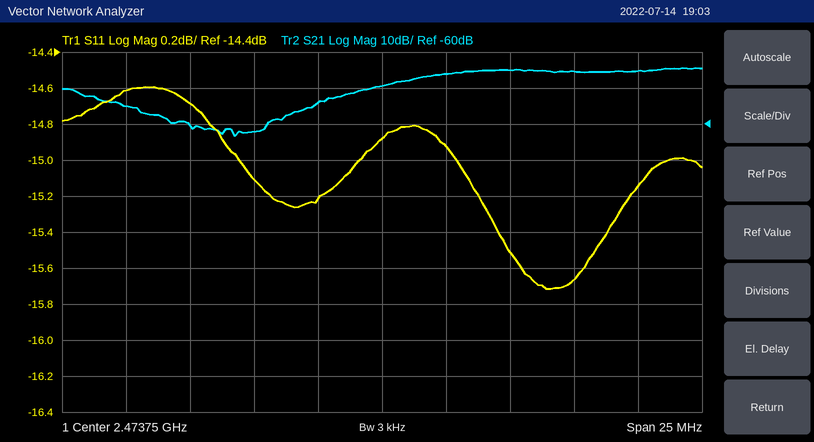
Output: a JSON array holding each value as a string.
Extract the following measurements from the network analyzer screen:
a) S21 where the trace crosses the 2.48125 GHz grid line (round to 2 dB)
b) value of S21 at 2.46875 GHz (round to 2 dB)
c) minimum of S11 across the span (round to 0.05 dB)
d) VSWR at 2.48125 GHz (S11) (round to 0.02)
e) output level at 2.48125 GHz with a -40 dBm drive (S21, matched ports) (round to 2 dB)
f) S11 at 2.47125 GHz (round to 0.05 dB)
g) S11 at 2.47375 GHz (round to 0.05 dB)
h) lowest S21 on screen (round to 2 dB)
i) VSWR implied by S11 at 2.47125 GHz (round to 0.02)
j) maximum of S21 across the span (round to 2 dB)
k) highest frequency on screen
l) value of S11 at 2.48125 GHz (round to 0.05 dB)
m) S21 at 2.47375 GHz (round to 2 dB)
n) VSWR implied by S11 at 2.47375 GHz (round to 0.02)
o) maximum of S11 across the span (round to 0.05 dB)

["-46 dB", "-62 dB", "-15.70 dB", "1.40", "-86 dBm", "-15.20 dB", "-14.90 dB", "-64 dB", "1.42", "-44 dB", "2.48625 GHz", "-15.65 dB", "-50 dB", "1.44", "-14.60 dB"]
